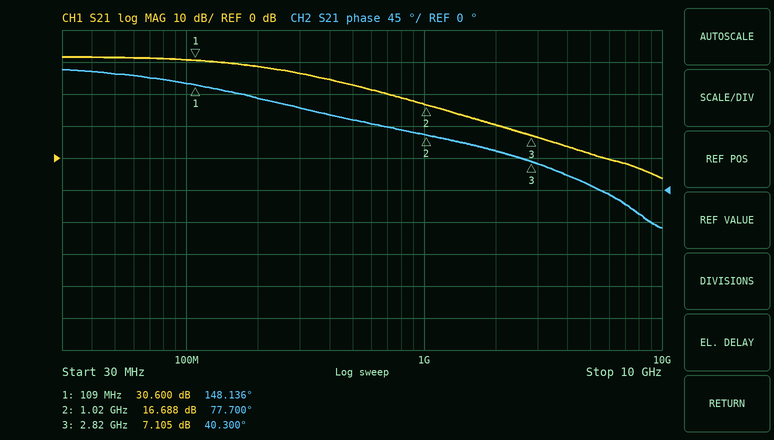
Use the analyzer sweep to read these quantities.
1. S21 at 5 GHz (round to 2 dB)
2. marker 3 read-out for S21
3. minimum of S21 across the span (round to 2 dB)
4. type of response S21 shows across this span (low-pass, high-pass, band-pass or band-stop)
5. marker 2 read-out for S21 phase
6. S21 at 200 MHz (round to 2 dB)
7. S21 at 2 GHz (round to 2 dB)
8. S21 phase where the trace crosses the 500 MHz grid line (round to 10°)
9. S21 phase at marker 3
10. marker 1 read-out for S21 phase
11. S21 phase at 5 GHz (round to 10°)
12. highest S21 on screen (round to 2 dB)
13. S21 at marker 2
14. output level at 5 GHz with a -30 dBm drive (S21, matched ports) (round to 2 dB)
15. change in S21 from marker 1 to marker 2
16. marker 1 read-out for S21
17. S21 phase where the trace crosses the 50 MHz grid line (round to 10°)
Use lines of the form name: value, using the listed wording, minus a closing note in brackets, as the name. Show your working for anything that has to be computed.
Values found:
S21 at 5 GHz: 2 dB
marker 3 read-out for S21: 7.105 dB
minimum of S21 across the span: -6 dB
type of response S21 shows across this span: low-pass
marker 2 read-out for S21 phase: 77.700°
S21 at 200 MHz: 28 dB
S21 at 2 GHz: 10 dB
S21 phase where the trace crosses the 500 MHz grid line: 100°
S21 phase at marker 3: 40.300°
marker 1 read-out for S21 phase: 148.136°
S21 phase at 5 GHz: 10°
highest S21 on screen: 32 dB
S21 at marker 2: 16.688 dB
output level at 5 GHz with a -30 dBm drive (S21, matched ports): -30 dBm + (2 dB) = -28 dBm
change in S21 from marker 1 to marker 2: 16.688 − (30.6) = -13.912 dB
marker 1 read-out for S21: 30.600 dB
S21 phase where the trace crosses the 50 MHz grid line: 160°
